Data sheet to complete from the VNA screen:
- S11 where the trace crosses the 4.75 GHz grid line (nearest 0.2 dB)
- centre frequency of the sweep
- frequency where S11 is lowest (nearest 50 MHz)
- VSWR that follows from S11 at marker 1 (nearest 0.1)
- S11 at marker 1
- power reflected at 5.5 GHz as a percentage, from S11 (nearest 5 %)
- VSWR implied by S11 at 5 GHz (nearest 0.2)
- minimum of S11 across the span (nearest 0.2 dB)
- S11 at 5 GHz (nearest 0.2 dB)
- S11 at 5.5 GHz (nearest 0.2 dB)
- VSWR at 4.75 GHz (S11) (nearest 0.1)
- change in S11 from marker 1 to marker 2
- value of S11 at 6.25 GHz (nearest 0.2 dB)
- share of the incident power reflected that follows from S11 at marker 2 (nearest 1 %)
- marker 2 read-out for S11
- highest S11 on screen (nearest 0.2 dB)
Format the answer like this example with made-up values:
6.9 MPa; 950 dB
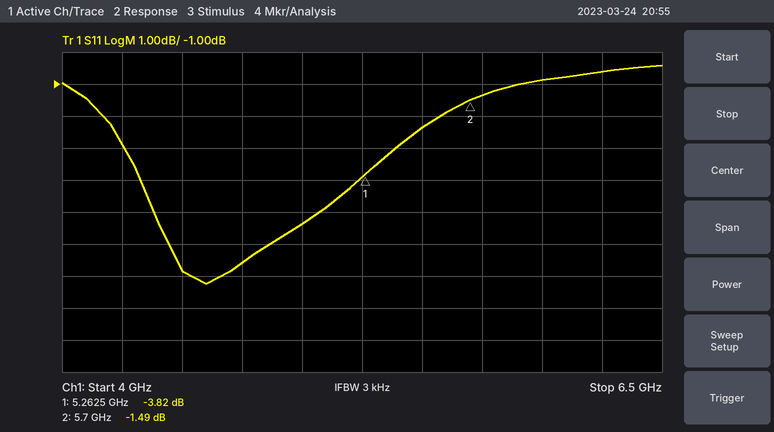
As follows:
-6.6 dB; 5.25 GHz; 4.60 GHz; 4.6; -3.82 dB; 60 %; 3.4; -7.2 dB; -5.4 dB; -2.4 dB; 2.8; 2.33 dB; -0.6 dB; 71 %; -1.49 dB; -0.4 dB
